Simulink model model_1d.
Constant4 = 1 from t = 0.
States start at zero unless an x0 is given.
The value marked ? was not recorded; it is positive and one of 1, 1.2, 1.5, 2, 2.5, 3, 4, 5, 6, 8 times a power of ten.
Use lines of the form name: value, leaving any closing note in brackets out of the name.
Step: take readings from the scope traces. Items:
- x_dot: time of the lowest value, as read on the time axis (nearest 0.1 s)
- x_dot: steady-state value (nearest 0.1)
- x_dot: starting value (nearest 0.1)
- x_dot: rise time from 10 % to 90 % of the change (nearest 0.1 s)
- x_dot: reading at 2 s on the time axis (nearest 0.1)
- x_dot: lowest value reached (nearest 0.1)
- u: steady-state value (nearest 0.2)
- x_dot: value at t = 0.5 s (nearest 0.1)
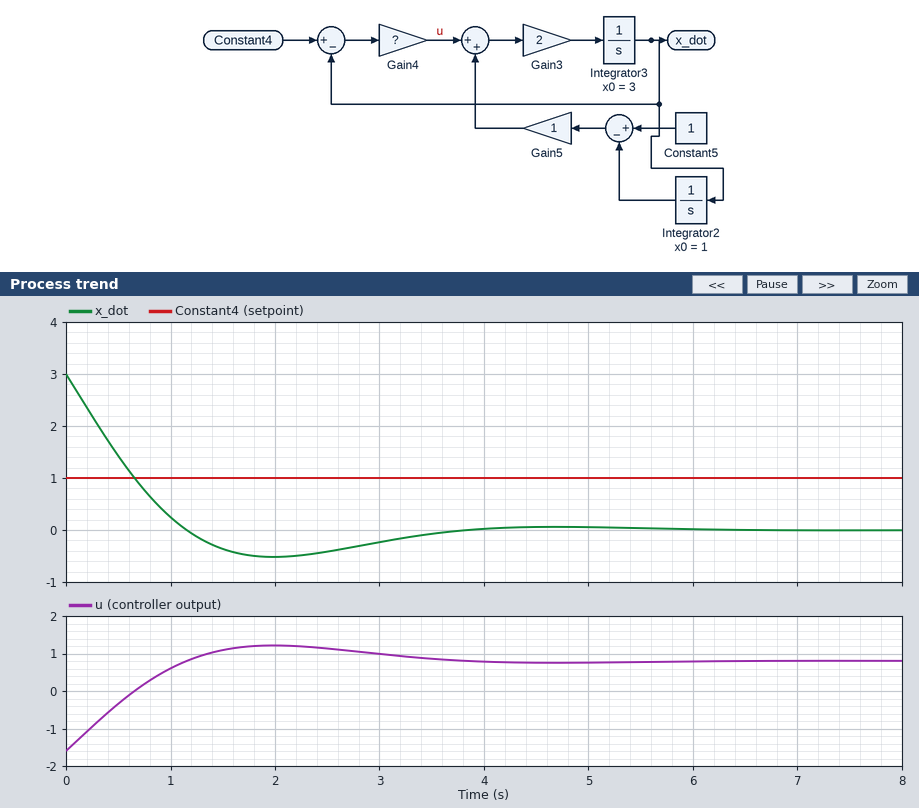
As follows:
x_dot: time of the lowest value, as read on the time axis: 2.0 s
x_dot: steady-state value: 0.0
x_dot: starting value: 3.0
x_dot: rise time from 10 % to 90 % of the change: 0.9 s
x_dot: reading at 2 s on the time axis: -0.5
x_dot: lowest value reached: -0.5
u: steady-state value: 0.8
x_dot: value at t = 0.5 s: 1.4
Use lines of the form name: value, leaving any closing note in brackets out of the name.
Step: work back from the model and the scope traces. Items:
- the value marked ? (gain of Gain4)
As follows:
the value marked ?: 0.8
